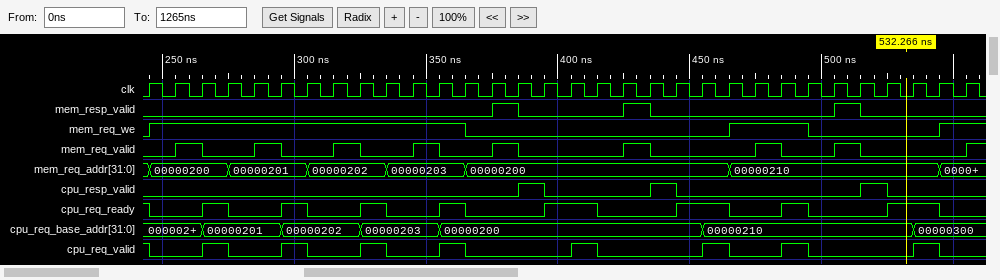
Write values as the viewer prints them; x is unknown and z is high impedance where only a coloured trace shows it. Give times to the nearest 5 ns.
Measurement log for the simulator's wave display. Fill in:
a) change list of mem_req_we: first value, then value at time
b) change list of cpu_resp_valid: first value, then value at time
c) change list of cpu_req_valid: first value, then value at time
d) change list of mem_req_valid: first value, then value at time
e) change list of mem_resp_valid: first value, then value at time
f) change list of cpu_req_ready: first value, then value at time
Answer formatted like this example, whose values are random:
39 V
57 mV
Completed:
0, 1 at 245 ns, 0 at 365 ns, 1 at 465 ns, 0 at 495 ns, 1 at 545 ns
0, 1 at 385 ns, 0 at 395 ns, 1 at 435 ns, 0 at 445 ns, 1 at 515 ns, 0 at 525 ns
1, 0 at 245 ns, 1 at 265 ns, 0 at 275 ns, 1 at 295 ns, 0 at 305 ns, 1 at 325 ns, 0 at 335 ns, 1 at 355 ns, 0 at 365 ns, 1 at 405 ns, 0 at 415 ns, 1 at 455 ns, 0 at 465 ns, 1 at 485 ns, 0 at 495 ns, 1 at 535 ns, 0 at 545 ns
0, 1 at 255 ns, 0 at 265 ns, 1 at 285 ns, 0 at 295 ns, 1 at 315 ns, 0 at 325 ns, 1 at 345 ns, 0 at 355 ns, 1 at 375 ns, 0 at 385 ns, 1 at 425 ns, 0 at 435 ns, 1 at 475 ns, 0 at 485 ns, 1 at 505 ns, 0 at 515 ns, 1 at 555 ns
0, 1 at 375 ns, 0 at 385 ns, 1 at 425 ns, 0 at 435 ns, 1 at 505 ns, 0 at 515 ns
1, 0 at 245 ns, 1 at 265 ns, 0 at 275 ns, 1 at 295 ns, 0 at 305 ns, 1 at 325 ns, 0 at 335 ns, 1 at 355 ns, 0 at 365 ns, 1 at 395 ns, 0 at 415 ns, 1 at 445 ns, 0 at 465 ns, 1 at 485 ns, 0 at 495 ns, 1 at 525 ns, 0 at 545 ns
